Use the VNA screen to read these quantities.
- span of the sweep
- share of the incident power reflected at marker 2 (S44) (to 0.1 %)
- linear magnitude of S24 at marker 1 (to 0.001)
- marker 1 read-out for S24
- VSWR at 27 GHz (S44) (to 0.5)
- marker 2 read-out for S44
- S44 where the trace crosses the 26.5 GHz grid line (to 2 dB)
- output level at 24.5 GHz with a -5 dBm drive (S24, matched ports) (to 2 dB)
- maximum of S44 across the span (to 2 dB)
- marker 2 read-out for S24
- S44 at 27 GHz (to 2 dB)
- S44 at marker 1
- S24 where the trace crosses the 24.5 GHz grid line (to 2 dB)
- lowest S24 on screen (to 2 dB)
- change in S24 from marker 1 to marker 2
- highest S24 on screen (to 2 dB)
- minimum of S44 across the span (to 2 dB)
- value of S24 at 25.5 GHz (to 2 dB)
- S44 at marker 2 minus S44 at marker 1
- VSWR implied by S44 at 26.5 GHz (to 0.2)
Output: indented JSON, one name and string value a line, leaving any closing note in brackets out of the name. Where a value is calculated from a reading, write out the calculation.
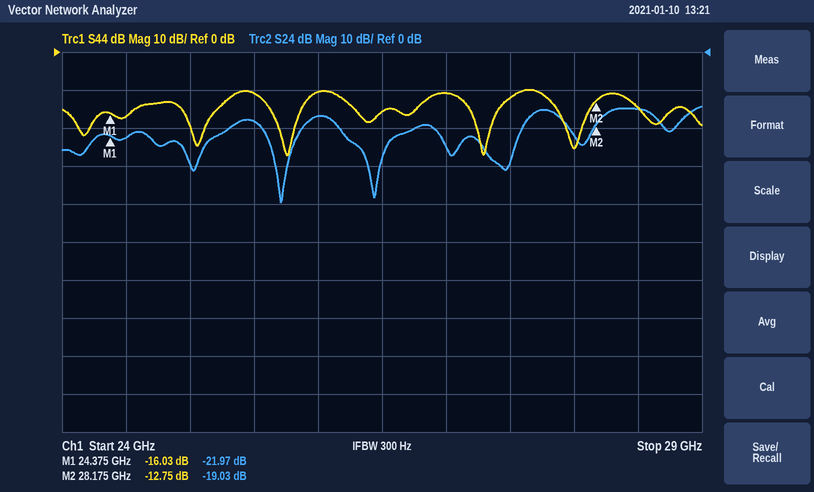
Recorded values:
{
  "span of the sweep": "5 GHz",
  "share of the incident power reflected at marker 2 (S44)": "10^(-12.75/10) ≈ 5.3 %",
  "linear magnitude of S24 at marker 1": "10^(-21.97/20) ≈ 0.080",
  "marker 1 read-out for S24": "-21.97 dB",
  "VSWR at 27 GHz (S44)": "|Γ| = 10^(-10/20) = 0.3162; VSWR = (1 + 0.3162)/(1 − 0.3162) ≈ 1.92, so 2.0 to the nearest 0.5",
  "marker 2 read-out for S44": "-12.75 dB",
  "S44 where the trace crosses the 26.5 GHz grid line": "-16 dB",
  "output level at 24.5 GHz with a -5 dBm drive (S24, matched ports)": "-5 dBm + (-22 dB) = -28 dBm",
  "maximum of S44 across the span": "-10 dB",
  "marker 2 read-out for S24": "-19.03 dB",
  "S44 at 27 GHz": "-10 dB",
  "S44 at marker 1": "-16.03 dB",
  "S24 where the trace crosses the 24.5 GHz grid line": "-22 dB",
  "lowest S24 on screen": "-40 dB",
  "change in S24 from marker 1 to marker 2": "-19.03 − (-21.97) = 2.94 dB",
  "highest S24 on screen": "-14 dB",
  "minimum of S44 across the span": "-28 dB",
  "value of S24 at 25.5 GHz": "-18 dB",
  "S44 at marker 2 minus S44 at marker 1": "-12.75 − (-16.03) = 3.28 dB",
  "VSWR implied by S44 at 26.5 GHz": "|Γ| = 10^(-16/20) = 0.1585; VSWR = (1 + 0.1585)/(1 − 0.1585) ≈ 1.4"
}
